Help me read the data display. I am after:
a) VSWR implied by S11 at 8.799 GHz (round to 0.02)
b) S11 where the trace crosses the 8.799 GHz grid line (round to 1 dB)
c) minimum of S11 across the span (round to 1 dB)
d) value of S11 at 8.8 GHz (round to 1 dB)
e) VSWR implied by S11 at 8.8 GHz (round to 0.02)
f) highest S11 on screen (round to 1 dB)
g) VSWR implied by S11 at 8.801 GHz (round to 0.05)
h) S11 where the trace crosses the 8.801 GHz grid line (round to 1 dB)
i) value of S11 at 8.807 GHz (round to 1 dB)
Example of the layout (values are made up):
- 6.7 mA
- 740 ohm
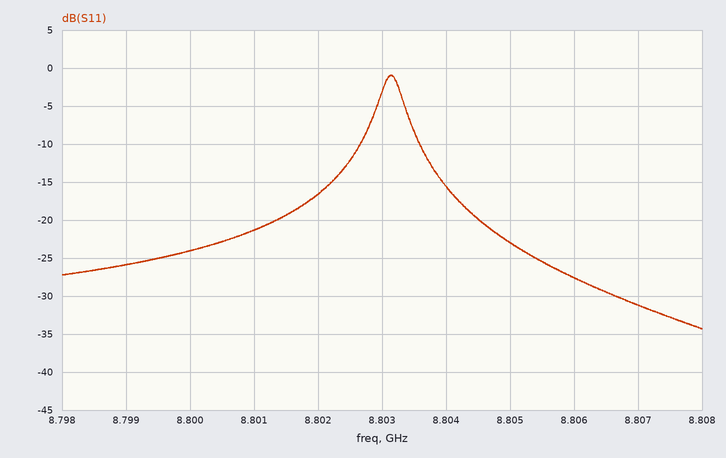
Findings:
- 1.10
- -26 dB
- -34 dB
- -24 dB
- 1.14
- -1 dB
- 1.20
- -21 dB
- -31 dB
